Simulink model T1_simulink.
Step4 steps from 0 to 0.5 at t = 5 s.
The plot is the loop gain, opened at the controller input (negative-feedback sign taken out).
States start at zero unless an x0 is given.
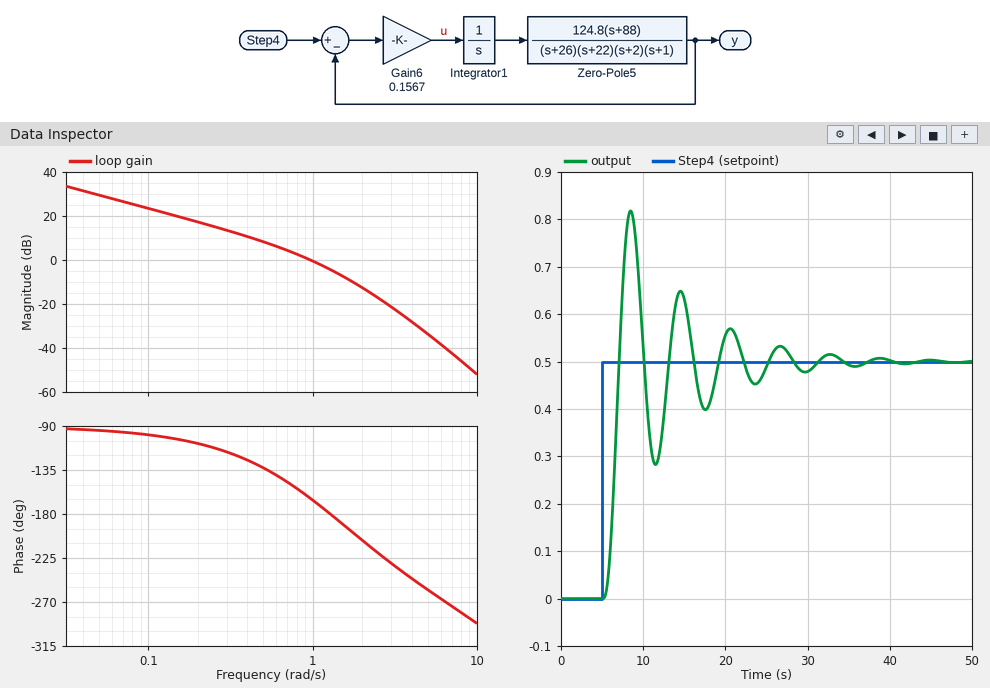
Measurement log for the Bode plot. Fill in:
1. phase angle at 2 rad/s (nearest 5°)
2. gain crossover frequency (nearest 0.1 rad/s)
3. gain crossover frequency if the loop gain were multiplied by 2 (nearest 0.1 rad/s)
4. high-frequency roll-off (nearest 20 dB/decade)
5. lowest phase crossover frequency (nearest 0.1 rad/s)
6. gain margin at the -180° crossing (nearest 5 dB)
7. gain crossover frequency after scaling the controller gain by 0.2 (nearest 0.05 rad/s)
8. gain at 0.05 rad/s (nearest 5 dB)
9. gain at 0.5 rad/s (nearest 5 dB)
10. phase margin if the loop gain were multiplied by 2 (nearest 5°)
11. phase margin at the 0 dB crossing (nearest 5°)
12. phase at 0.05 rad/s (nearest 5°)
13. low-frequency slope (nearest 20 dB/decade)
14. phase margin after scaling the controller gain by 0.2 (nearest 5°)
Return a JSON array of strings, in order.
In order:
["-205°", "1.0 rad/s", "1.4 rad/s", "-60 dB/decade", "1.3 rad/s", "5 dB", "0.30 rad/s", "30 dB", "10 dB", "-5°", "15°", "-95°", "-20 dB/decade", "65°"]
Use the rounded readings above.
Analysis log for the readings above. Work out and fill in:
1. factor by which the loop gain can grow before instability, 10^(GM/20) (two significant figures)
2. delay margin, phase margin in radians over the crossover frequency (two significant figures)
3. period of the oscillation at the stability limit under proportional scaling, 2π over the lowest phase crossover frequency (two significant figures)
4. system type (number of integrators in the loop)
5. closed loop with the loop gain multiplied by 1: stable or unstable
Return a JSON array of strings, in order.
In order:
["1.8", "0.26 s", "4.8 s", "1", "stable"]
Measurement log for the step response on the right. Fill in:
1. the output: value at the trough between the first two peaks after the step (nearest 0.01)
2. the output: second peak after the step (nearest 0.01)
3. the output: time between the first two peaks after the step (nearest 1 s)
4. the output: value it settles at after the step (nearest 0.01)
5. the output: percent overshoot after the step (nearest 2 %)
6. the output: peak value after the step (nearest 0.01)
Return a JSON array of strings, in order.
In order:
["0.28", "0.65", "6 s", "0.50", "64 %", "0.82"]
